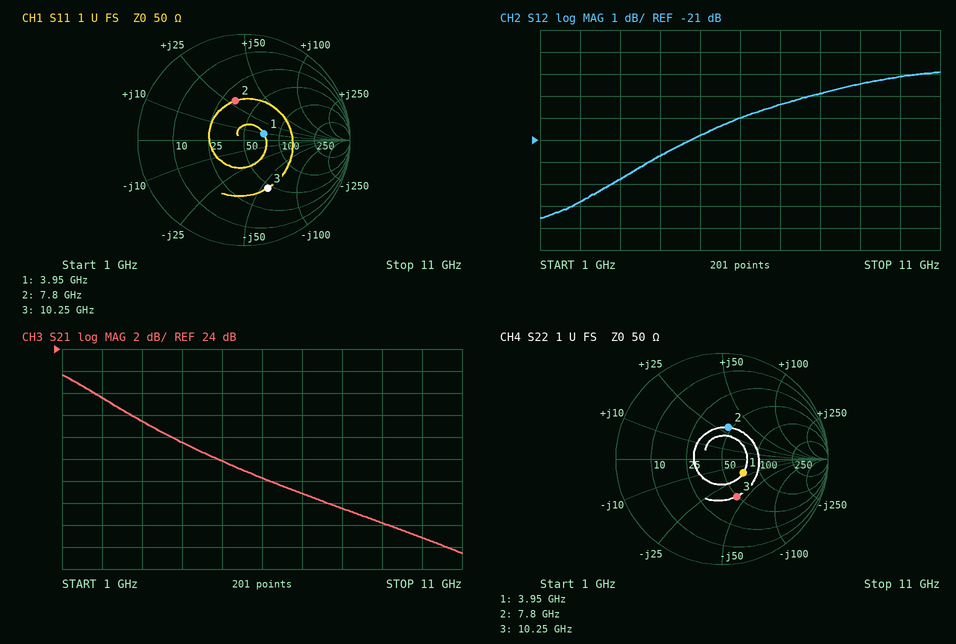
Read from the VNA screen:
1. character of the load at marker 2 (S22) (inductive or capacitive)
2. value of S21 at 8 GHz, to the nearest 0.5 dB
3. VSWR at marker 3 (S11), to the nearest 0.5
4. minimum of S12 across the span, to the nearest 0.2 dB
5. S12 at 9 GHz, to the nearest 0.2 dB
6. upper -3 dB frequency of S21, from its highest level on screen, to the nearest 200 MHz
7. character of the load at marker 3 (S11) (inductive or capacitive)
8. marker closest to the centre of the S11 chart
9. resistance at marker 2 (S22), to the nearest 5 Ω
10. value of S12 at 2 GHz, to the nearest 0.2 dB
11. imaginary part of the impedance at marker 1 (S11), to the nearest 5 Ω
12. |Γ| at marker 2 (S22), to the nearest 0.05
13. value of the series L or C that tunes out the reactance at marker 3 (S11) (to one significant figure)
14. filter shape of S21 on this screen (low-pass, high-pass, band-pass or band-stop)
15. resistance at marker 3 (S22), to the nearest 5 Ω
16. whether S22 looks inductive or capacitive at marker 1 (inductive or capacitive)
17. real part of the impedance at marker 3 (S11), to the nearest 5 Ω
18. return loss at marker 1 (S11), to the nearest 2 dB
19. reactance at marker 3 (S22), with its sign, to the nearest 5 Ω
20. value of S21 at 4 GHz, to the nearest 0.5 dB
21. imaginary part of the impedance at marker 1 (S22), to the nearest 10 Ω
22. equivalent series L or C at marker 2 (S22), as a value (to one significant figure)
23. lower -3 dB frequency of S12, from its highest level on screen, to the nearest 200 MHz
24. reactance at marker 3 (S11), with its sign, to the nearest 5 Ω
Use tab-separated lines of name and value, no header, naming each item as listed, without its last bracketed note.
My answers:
character of the load at marker 2 (S22)	inductive
value of S21 at 8 GHz, to the nearest 0.5 dB	9.5 dB
VSWR at marker 3 (S11), to the nearest 0.5	3.0
minimum of S12 across the span, to the nearest 0.2 dB	-24.6 dB
S12 at 9 GHz, to the nearest 0.2 dB	-18.4 dB
upper -3 dB frequency of S21, from its highest level on screen, to the nearest 200 MHz	2.4 GHz
character of the load at marker 3 (S11)	capacitive
marker closest to the centre of the S11 chart	marker 1
resistance at marker 2 (S22), to the nearest 5 Ω	45 Ω
value of S12 at 2 GHz, to the nearest 0.2 dB	-23.8 dB
imaginary part of the impedance at marker 1 (S11), to the nearest 5 Ω	+10 Ω
|Γ| at marker 2 (S22), to the nearest 0.05	0.30
value of the series L or C that tunes out the reactance at marker 3 (S11)	900 pH
filter shape of S21 on this screen	low-pass
resistance at marker 3 (S22), to the nearest 5 Ω	50 Ω
whether S22 looks inductive or capacitive at marker 1	capacitive
real part of the impedance at marker 3 (S11), to the nearest 5 Ω	45 Ω
return loss at marker 1 (S11), to the nearest 2 dB	14 dB
reactance at marker 3 (S22), with its sign, to the nearest 5 Ω	-40 Ω
value of S21 at 4 GHz, to the nearest 0.5 dB	15.5 dB
imaginary part of the impedance at marker 1 (S22), to the nearest 10 Ω	-20 Ω
equivalent series L or C at marker 2 (S22), as a value	600 pH
lower -3 dB frequency of S12, from its highest level on screen, to the nearest 200 MHz	4.8 GHz
reactance at marker 3 (S11), with its sign, to the nearest 5 Ω	-55 Ω
